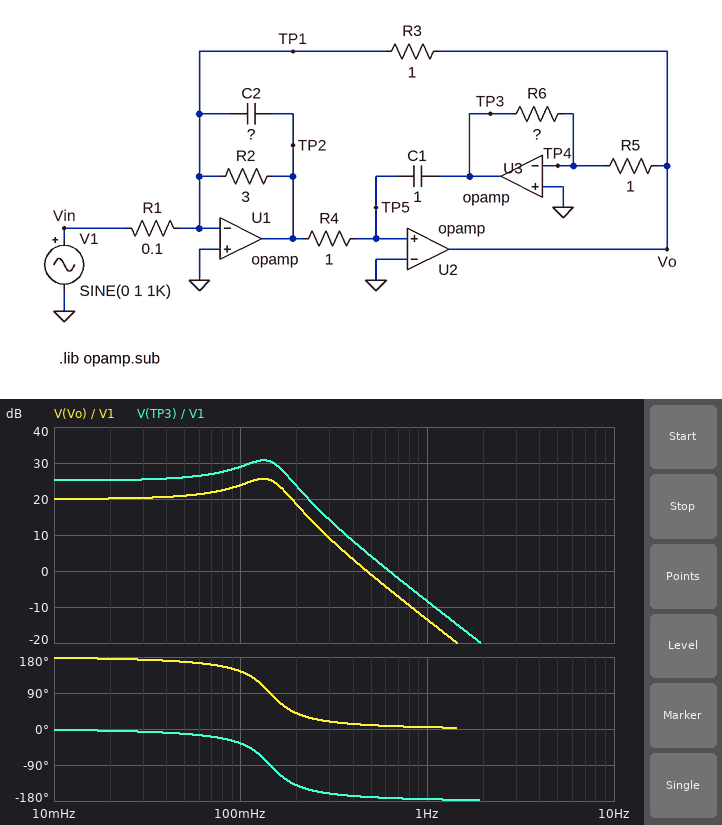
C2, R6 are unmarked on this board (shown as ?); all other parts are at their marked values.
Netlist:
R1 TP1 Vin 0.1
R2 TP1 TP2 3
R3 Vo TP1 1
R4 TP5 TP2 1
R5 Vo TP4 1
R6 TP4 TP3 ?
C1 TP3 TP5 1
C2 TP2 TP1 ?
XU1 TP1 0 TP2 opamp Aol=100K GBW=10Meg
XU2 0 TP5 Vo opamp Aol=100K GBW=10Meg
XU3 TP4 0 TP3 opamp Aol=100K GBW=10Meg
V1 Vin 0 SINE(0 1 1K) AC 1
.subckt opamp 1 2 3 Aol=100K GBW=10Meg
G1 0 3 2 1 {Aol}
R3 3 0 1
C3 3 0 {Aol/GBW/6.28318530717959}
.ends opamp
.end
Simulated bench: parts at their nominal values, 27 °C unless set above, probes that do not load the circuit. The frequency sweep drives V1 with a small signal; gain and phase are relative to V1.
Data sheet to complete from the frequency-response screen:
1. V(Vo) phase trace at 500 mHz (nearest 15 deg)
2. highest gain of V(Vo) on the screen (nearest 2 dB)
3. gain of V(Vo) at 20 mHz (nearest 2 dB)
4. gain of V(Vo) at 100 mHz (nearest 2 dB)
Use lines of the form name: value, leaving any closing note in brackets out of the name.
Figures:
V(Vo) phase trace at 500 mHz: 15 deg
highest gain of V(Vo) on the screen: 26 dB
gain of V(Vo) at 20 mHz: 20 dB
gain of V(Vo) at 100 mHz: 24 dB
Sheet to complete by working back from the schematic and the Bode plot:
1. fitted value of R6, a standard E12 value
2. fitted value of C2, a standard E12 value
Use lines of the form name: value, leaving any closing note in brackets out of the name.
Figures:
fitted value of R6, a standard E12 value: 1.8 Ω
fitted value of C2, a standard E12 value: 680 mF
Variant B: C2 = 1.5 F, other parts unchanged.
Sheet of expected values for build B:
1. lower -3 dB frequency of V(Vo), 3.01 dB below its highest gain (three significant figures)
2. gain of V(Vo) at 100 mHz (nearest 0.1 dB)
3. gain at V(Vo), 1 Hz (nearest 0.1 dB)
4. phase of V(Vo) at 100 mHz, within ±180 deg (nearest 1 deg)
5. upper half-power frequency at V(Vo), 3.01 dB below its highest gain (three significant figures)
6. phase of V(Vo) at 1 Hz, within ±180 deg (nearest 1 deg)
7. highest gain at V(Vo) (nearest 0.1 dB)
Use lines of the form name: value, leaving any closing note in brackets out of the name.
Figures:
lower -3 dB frequency of V(Vo), 3.01 dB below its highest gain: 73.4 mHz
gain of V(Vo) at 100 mHz: 28.3 dB
gain at V(Vo), 1 Hz: -20.5 dB
phase of V(Vo) at 100 mHz, within ±180 deg: 80 deg
upper half-power frequency at V(Vo), 3.01 dB below its highest gain: 110 mHz
phase of V(Vo) at 1 Hz, within ±180 deg: 2 deg
highest gain at V(Vo): 28.9 dB
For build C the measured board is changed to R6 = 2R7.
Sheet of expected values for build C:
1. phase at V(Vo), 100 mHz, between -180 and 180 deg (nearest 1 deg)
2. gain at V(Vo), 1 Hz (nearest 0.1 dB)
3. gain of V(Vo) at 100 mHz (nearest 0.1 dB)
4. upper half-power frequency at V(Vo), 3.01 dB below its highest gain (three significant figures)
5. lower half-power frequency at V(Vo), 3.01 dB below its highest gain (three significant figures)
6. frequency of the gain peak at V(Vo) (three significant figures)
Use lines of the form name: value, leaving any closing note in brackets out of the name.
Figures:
phase at V(Vo), 100 mHz, between -180 and 180 deg: 116 deg
gain at V(Vo), 1 Hz: -17.1 dB
gain of V(Vo) at 100 mHz: 24.0 dB
upper half-power frequency at V(Vo), 3.01 dB below its highest gain: 139 mHz
lower half-power frequency at V(Vo), 3.01 dB below its highest gain: 45.8 mHz
frequency of the gain peak at V(Vo): 104 mHz
